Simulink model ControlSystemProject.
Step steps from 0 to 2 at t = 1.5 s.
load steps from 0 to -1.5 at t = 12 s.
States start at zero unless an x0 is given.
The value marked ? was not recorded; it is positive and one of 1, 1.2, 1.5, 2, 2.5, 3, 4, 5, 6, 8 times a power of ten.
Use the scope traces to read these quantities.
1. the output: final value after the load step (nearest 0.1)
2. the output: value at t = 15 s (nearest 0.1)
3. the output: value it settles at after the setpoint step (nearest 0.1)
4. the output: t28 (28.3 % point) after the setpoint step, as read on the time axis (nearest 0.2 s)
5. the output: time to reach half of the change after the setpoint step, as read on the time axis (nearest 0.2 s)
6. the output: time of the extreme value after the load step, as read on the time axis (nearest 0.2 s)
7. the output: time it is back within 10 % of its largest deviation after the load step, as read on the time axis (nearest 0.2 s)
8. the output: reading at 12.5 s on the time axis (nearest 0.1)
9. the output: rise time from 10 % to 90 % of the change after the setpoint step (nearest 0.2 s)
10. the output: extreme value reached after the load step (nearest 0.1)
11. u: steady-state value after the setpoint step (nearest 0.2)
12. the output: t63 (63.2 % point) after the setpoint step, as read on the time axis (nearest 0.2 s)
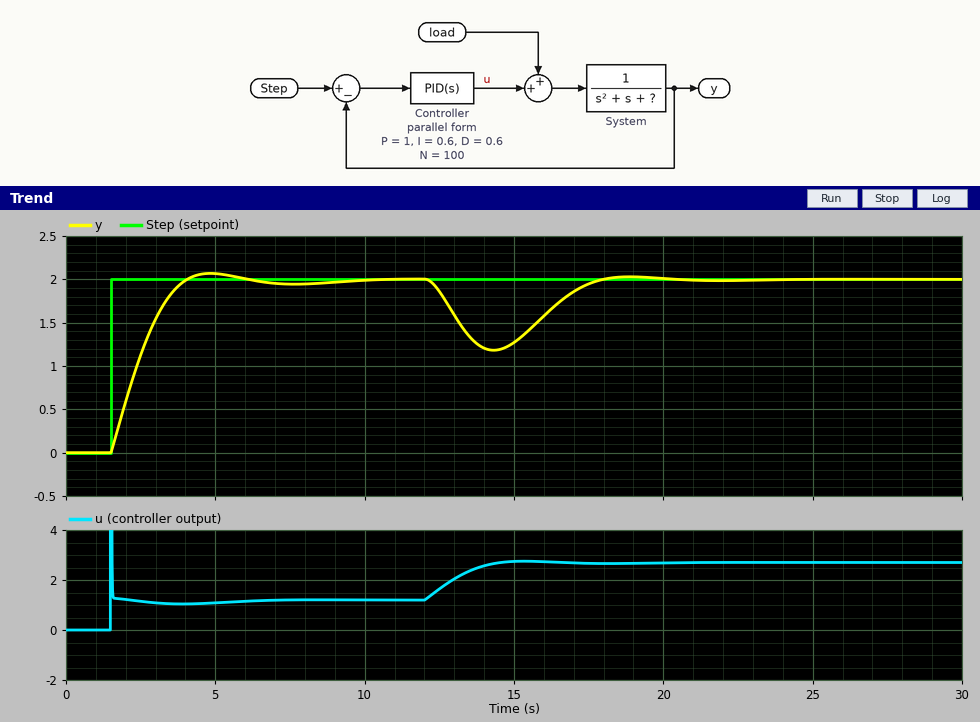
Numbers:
2.0
1.3
2.0
2.0 s
2.4 s
14.4 s
17.4 s
1.9
1.8 s
1.2
1.2
2.6 s
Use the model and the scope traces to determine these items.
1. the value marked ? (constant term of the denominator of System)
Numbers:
0.6
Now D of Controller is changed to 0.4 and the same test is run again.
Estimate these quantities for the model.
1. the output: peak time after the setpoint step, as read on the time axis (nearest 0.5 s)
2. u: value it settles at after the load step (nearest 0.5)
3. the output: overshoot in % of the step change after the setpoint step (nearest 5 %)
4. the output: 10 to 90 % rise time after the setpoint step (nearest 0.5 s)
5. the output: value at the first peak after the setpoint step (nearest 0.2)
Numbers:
4.5 s
2.5
10 %
1.5 s
2.2
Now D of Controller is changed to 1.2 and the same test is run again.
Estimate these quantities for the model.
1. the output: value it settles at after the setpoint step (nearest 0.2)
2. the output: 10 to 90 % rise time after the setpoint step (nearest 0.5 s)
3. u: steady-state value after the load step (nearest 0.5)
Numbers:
2.0
2.5 s
2.5
